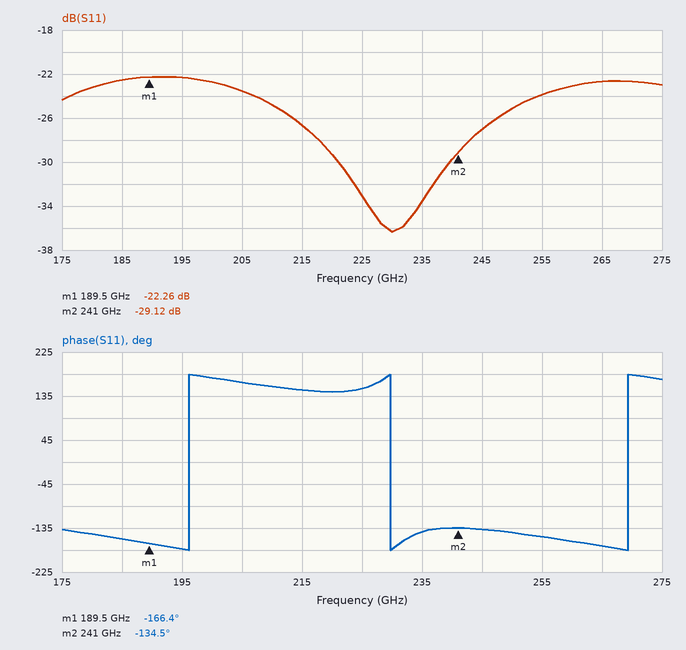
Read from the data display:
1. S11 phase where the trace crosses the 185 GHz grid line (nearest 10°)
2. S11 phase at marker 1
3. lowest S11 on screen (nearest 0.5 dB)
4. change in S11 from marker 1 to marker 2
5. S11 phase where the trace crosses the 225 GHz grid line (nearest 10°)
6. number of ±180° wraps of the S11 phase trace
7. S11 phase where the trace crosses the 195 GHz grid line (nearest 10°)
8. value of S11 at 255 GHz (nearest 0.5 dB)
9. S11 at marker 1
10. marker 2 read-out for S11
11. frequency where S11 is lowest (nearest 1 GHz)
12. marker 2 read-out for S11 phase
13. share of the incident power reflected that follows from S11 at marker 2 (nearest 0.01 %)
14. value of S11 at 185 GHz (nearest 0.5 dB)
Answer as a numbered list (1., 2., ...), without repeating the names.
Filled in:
1. -160°
2. -166.4°
3. -36.5 dB
4. -6.86 dB
5. 150°
6. 3
7. -180°
8. -24.0 dB
9. -22.26 dB
10. -29.12 dB
11. 230 GHz
12. -134.5°
13. 0.12 %
14. -22.5 dB
